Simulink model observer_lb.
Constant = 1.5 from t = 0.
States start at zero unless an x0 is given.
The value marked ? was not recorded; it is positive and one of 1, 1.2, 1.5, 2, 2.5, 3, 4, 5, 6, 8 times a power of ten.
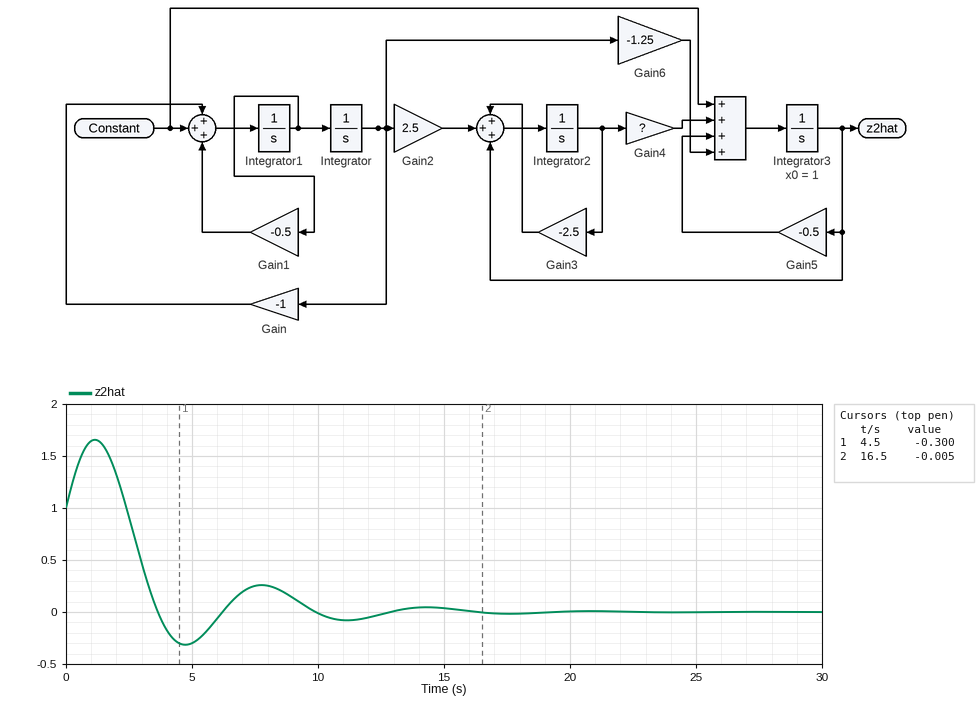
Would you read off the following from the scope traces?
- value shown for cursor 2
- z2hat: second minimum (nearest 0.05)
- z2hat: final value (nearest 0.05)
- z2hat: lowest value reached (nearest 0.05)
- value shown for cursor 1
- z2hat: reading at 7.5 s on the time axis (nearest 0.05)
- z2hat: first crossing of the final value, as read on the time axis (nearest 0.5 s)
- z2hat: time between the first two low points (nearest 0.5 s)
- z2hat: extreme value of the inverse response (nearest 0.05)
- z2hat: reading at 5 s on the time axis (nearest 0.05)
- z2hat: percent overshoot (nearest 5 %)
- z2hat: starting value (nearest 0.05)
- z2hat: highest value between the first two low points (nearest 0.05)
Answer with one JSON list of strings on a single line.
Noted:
["-0.005", "-0.10", "0.00", "-0.30", "-0.300", "0.25", "3.5 s", "6.5 s", "1.65", "-0.30", "30 %", "1.00", "0.25"]
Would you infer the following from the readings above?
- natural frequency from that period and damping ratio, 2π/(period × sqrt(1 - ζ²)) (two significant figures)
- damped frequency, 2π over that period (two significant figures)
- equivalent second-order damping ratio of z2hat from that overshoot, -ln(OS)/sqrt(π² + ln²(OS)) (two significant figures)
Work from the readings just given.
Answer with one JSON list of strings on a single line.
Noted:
["1.0 rad/s", "0.97 rad/s", "0.36"]
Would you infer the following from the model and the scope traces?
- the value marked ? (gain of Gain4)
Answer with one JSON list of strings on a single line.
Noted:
["0.25"]
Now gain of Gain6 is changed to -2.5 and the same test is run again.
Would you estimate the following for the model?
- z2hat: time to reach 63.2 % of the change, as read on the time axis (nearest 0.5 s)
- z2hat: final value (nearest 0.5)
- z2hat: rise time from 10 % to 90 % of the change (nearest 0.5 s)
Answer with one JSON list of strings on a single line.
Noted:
["3.0 s", "-4.5", "2.0 s"]
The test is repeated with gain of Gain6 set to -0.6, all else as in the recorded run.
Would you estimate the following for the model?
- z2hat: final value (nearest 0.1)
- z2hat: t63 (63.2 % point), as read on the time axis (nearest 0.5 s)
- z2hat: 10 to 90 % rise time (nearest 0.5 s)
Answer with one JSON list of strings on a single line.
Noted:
["2.4", "1.5 s", "6.0 s"]
